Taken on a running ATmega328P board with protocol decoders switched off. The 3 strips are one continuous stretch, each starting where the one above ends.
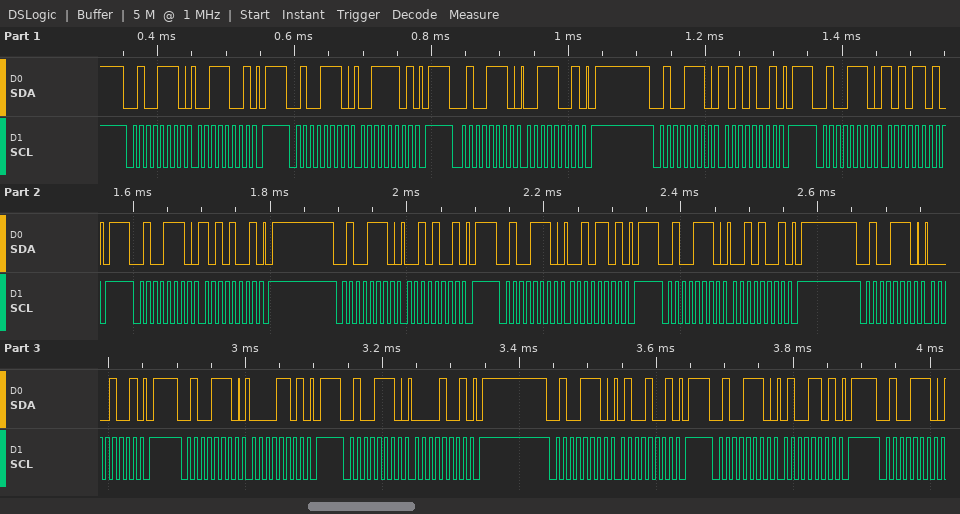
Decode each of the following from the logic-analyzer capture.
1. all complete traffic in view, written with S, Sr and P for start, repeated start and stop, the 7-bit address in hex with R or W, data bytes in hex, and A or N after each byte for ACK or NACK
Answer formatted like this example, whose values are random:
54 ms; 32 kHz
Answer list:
S 27W A 39 A P S 27W A 3D A P S 27W A 39 A P S 27W A A9 A P S 27W A AD A P S 27W A A9 A P S 27W A 29 A P S 27W A 2D A P S 27W A 29 A P S 27W A 09 A P S 27W A 0D A P S 27W A 09 A P S 27W A 49 A P S 27W A 4D A P S 27W A
